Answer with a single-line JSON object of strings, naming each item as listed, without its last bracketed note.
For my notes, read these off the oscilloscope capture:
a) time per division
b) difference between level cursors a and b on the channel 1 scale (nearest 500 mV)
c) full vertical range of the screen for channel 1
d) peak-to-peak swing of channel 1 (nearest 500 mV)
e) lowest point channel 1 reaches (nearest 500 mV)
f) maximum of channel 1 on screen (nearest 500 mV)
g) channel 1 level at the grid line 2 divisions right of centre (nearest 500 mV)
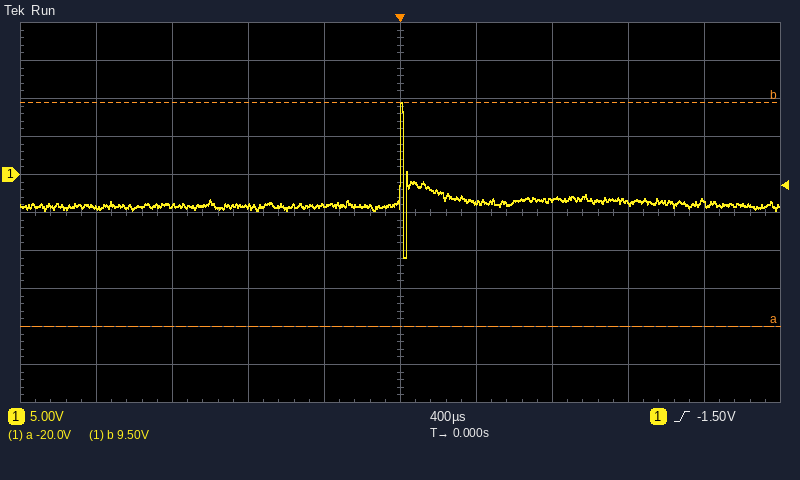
{"time per division": "400 µs", "difference between level cursors a and b on the channel 1 scale": "29.5 V", "full vertical range of the screen for channel 1": "50 V", "peak-to-peak swing of channel 1": "20.5 V", "lowest point channel 1 reaches": "-11.0 V", "maximum of channel 1 on screen": "9.5 V", "channel 1 level at the grid line 2 divisions right of centre": "-3.5 V"}
